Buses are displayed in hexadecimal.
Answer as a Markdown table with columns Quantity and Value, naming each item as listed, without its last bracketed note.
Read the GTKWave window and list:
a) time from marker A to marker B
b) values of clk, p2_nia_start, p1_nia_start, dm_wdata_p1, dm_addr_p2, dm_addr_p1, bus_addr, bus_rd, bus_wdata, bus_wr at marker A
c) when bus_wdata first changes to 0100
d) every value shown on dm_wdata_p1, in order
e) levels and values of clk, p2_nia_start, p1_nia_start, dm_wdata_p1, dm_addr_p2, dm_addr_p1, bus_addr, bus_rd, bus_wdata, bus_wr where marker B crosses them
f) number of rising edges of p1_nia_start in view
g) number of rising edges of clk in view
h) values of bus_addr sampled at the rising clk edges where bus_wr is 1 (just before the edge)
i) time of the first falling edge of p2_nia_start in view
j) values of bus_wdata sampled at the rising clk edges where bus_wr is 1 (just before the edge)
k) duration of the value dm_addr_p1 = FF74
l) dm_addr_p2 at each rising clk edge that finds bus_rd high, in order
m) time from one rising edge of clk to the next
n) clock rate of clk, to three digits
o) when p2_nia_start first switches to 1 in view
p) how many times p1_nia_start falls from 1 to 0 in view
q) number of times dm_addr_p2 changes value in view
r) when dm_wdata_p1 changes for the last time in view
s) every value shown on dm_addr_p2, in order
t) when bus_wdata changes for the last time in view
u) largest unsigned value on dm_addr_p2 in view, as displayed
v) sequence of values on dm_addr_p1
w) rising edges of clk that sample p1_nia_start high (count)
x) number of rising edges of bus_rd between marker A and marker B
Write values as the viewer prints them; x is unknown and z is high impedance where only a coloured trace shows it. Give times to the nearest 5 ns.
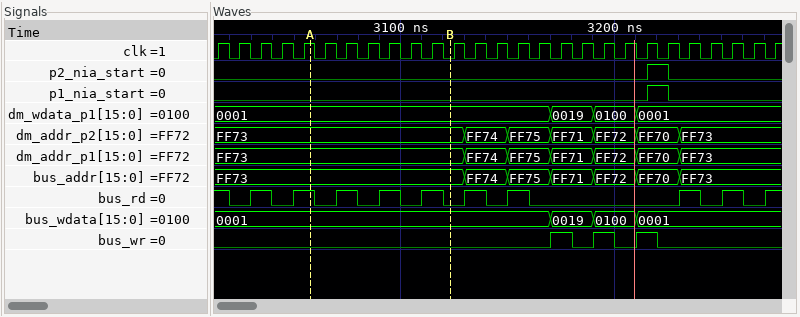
| Quantity | Value |
|---|---|
| time from marker A to marker B | 65 ns |
| values of clk, p2_nia_start, p1_nia_start, dm_wdata_p1, dm_addr_p2, dm_addr_p1, bus_addr, bus_rd, bus_wdata, bus_wr at marker A | clk=1, p2_nia_start=0, p1_nia_start=0, dm_wdata_p1=0001, dm_addr_p2=FF73, dm_addr_p1=FF73, bus_addr=FF73, bus_rd=1, bus_wdata=0001, bus_wr=0 |
| when bus_wdata first changes to 0100 | 3190 ns |
| every value shown on dm_wdata_p1, in order | 0001, 0019, 0100, 0001 |
| levels and values of clk, p2_nia_start, p1_nia_start, dm_wdata_p1, dm_addr_p2, dm_addr_p1, bus_addr, bus_rd, bus_wdata, bus_wr where marker B crosses them | clk=0, p2_nia_start=0, p1_nia_start=0, dm_wdata_p1=0001, dm_addr_p2=FF73, dm_addr_p1=FF73, bus_addr=FF73, bus_rd=0, bus_wdata=0001, bus_wr=0 |
| number of rising edges of p1_nia_start in view | 1 |
| number of rising edges of clk in view | 27 |
| values of bus_addr sampled at the rising clk edges where bus_wr is 1 | FF71, FF72, FF70 |
| time of the first falling edge of p2_nia_start in view | 3225 ns |
| values of bus_wdata sampled at the rising clk edges where bus_wr is 1 | 0019, 0100, 0001 |
| duration of the value dm_addr_p1 = FF74 | 20 ns |
| dm_addr_p2 at each rising clk edge that finds bus_rd high, in order | FF73, FF73, FF73, FF73, FF73, FF73, FF74, FF75, FF73, FF73, FF73 |
| time from one rising edge of clk to the next | 10 ns |
| clock rate of clk, to three digits | 100 MHz |
| when p2_nia_start first switches to 1 in view | 3215 ns |
| how many times p1_nia_start falls from 1 to 0 in view | 1 |
| number of times dm_addr_p2 changes value in view | 6 |
| when dm_wdata_p1 changes for the last time in view | 3210 ns |
| every value shown on dm_addr_p2, in order | FF73, FF74, FF75, FF71, FF72, FF70, FF73 |
| when bus_wdata changes for the last time in view | 3210 ns |
| largest unsigned value on dm_addr_p2 in view, as displayed | FF75 |
| sequence of values on dm_addr_p1 | FF73, FF74, FF75, FF71, FF72, FF70, FF73 |
| rising edges of clk that sample p1_nia_start high | 1 |
| number of rising edges of bus_rd between marker A and marker B | 3 |
